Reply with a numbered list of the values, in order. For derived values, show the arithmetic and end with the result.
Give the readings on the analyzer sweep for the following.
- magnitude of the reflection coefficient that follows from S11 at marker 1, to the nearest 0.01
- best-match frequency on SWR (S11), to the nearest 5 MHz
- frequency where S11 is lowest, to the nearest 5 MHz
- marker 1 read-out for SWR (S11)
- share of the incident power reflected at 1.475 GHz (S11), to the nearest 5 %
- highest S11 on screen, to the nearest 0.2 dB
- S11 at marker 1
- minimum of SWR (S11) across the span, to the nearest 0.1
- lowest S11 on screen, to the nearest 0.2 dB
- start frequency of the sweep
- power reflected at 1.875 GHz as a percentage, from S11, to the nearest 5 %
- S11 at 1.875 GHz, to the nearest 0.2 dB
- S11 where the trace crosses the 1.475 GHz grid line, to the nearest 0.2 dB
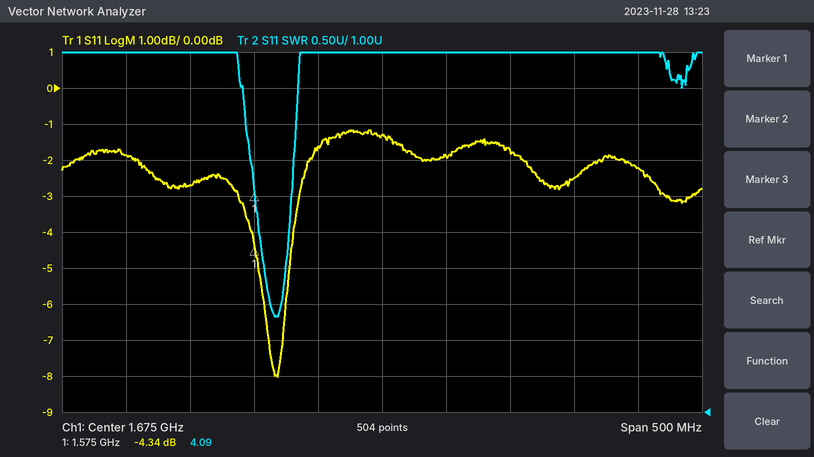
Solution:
1. 10^(-4.34/20) ≈ 0.61
2. 1.595 GHz
3. 1.595 GHz
4. 4.09
5. 10^(-1.8/10) ≈ 66.1 %, so 65 % to the nearest 5 %
6. -1.2 dB
7. -4.34 dB
8. 2.3
9. -8.0 dB
10. 1.425 GHz
11. 10^(-2.2/10) ≈ 60 %
12. -2.2 dB
13. -1.8 dB
